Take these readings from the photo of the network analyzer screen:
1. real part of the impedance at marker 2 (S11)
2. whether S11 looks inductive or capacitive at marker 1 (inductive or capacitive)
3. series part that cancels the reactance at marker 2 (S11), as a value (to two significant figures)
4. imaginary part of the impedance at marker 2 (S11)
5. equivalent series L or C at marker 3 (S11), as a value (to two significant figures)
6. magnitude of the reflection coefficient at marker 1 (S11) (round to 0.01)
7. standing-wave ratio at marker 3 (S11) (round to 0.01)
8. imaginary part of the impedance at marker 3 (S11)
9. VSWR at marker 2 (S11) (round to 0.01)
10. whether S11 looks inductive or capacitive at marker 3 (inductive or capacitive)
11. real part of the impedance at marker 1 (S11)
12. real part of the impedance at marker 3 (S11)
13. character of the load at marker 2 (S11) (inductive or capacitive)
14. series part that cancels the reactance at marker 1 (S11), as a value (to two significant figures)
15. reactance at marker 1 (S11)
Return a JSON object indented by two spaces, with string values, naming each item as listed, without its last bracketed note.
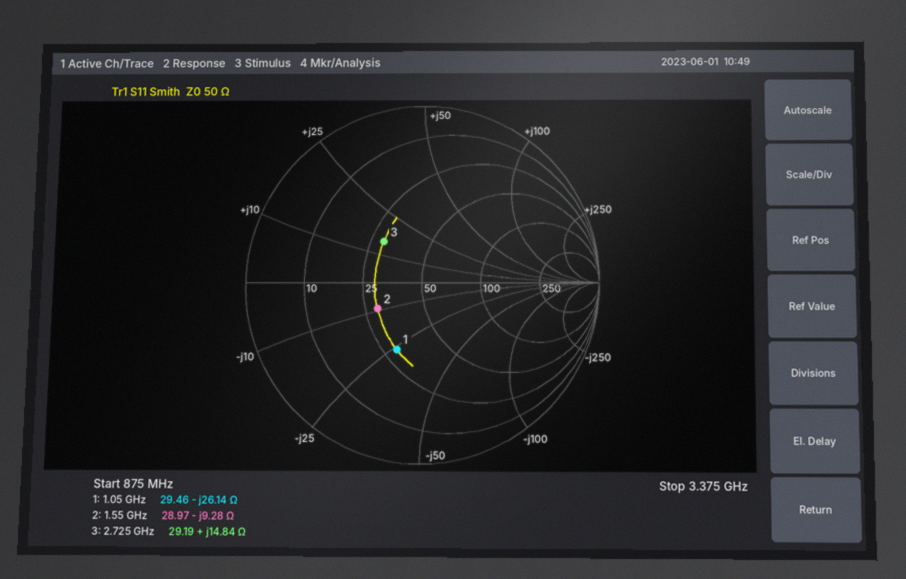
{
  "real part of the impedance at marker 2": "28.97 Ω",
  "whether S11 looks inductive or capacitive at marker 1": "capacitive",
  "series part that cancels the reactance at marker 2 (S11), as a value": "950 pH",
  "imaginary part of the impedance at marker 2": "-9.28 Ω",
  "equivalent series L or C at marker 3 (S11), as a value": "870 pH",
  "magnitude of the reflection coefficient at marker 1 (S11)": "0.40",
  "standing-wave ratio at marker 3 (S11)": "1.93",
  "imaginary part of the impedance at marker 3": "+14.84 Ω",
  "VSWR at marker 2 (S11)": "1.81",
  "whether S11 looks inductive or capacitive at marker 3": "inductive",
  "real part of the impedance at marker 1": "29.46 Ω",
  "real part of the impedance at marker 3": "29.19 Ω",
  "character of the load at marker 2 (S11)": "capacitive",
  "series part that cancels the reactance at marker 1 (S11), as a value": "4.0 nH",
  "reactance at marker 1": "-26.14 Ω"
}
